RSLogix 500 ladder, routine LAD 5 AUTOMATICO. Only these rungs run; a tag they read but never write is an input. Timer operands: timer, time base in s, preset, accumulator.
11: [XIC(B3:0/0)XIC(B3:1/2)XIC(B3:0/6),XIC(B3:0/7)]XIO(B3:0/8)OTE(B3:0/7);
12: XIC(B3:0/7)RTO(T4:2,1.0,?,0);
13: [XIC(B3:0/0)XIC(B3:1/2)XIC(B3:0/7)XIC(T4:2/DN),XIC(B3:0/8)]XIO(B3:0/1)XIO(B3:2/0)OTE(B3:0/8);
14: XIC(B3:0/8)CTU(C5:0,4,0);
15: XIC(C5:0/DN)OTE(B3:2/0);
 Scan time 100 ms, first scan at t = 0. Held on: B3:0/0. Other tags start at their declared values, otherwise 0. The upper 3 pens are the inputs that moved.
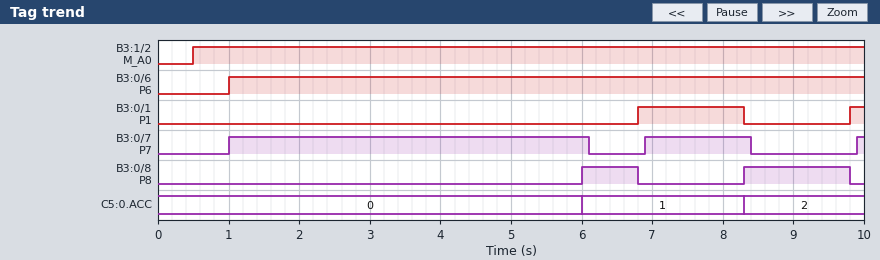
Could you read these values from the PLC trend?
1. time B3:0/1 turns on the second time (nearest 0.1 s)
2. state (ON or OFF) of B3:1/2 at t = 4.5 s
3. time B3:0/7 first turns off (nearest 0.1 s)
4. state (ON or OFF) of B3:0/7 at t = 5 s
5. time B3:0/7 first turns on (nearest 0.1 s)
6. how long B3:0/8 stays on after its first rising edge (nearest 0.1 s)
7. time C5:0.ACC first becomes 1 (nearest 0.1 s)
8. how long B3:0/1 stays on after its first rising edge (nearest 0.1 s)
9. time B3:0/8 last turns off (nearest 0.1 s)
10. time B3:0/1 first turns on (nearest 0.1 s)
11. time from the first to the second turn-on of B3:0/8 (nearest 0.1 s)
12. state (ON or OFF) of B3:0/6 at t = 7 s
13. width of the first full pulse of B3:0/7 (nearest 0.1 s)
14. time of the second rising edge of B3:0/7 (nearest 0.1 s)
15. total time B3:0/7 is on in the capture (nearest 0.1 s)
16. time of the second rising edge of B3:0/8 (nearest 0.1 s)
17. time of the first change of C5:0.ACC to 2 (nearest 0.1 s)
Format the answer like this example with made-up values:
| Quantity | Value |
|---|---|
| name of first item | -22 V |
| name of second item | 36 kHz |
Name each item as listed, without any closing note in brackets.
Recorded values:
| Quantity | Value |
|---|---|
| time B3:0/1 turns on the second time | 9.8 s |
| state (ON or OFF) of B3:1/2 at t = 4.5 s | ON |
| time B3:0/7 first turns off | 6.1 s |
| state (ON or OFF) of B3:0/7 at t = 5 s | ON |
| time B3:0/7 first turns on | 1.0 s |
| how long B3:0/8 stays on after its first rising edge | 0.8 s |
| time C5:0.ACC first becomes 1 | 6.0 s |
| how long B3:0/1 stays on after its first rising edge | 1.5 s |
| time B3:0/8 last turns off | 9.8 s |
| time B3:0/1 first turns on | 6.8 s |
| time from the first to the second turn-on of B3:0/8 | 2.3 s |
| state (ON or OFF) of B3:0/6 at t = 7 s | ON |
| width of the first full pulse of B3:0/7 | 5.1 s |
| time of the second rising edge of B3:0/7 | 6.9 s |
| total time B3:0/7 is on in the capture | 6.7 s |
| time of the second rising edge of B3:0/8 | 8.3 s |
| time of the first change of C5:0.ACC to 2 | 8.3 s |
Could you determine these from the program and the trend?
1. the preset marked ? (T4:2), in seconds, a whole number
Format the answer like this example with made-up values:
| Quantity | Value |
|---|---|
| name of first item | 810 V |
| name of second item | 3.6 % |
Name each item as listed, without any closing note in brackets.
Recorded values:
| Quantity | Value |
|---|---|
| the preset marked ? (T4:2), in seconds, a whole number | 5 s |
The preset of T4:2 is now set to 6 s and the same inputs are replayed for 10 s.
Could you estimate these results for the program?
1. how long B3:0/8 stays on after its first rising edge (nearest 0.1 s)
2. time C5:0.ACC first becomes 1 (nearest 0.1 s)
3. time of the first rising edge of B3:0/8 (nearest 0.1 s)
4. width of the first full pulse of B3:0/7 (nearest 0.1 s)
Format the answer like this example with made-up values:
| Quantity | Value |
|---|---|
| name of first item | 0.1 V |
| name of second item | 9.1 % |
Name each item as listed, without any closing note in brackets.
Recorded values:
| Quantity | Value |
|---|---|
| how long B3:0/8 stays on after its first rising edge | 1.5 s |
| time C5:0.ACC first becomes 1 | 8.3 s |
| time of the first rising edge of B3:0/8 | 8.3 s |
| width of the first full pulse of B3:0/7 | 7.4 s |
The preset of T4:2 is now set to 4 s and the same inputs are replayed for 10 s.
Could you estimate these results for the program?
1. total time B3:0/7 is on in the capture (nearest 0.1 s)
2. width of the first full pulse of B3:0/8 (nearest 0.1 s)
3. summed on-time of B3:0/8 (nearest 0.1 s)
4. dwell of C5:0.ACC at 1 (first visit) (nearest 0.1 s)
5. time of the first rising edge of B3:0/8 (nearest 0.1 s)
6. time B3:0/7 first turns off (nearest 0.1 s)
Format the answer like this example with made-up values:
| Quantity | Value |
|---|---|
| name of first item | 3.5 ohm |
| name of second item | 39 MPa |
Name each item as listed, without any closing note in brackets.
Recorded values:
| Quantity | Value |
|---|---|
| total time B3:0/7 is on in the capture | 5.7 s |
| width of the first full pulse of B3:0/8 | 1.8 s |
| summed on-time of B3:0/8 | 3.3 s |
| dwell of C5:0.ACC at 1 (first visit) | 3.3 s |
| time of the first rising edge of B3:0/8 | 5.0 s |
| time B3:0/7 first turns off | 5.1 s |
